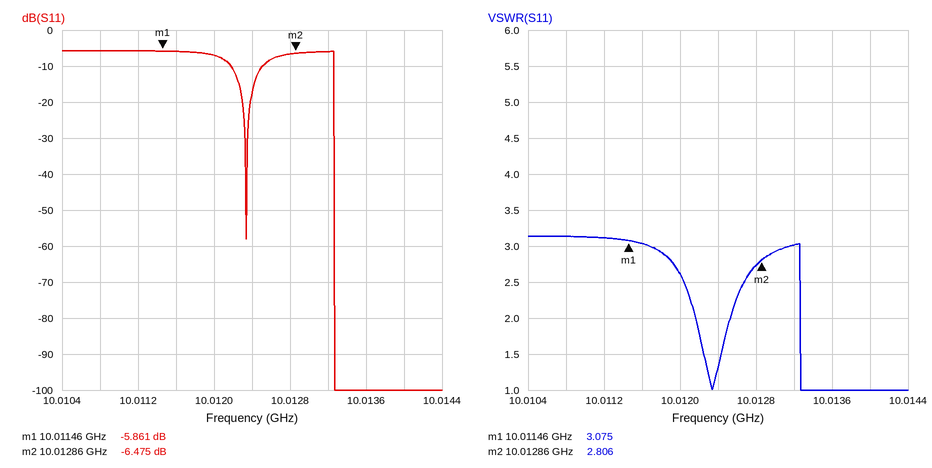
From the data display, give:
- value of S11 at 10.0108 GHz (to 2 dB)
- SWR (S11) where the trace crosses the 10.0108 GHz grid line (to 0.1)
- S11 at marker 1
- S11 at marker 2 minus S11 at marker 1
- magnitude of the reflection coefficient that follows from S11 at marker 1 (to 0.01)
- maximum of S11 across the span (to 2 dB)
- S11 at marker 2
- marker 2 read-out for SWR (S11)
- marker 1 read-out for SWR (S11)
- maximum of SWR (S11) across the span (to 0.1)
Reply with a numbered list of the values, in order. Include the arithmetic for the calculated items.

1. -6 dB
2. 3.1
3. -5.861 dB
4. -6.475 − (-5.861) = -0.614 dB
5. 10^(-5.861/20) ≈ 0.51
6. -6 dB
7. -6.475 dB
8. 2.806
9. 3.075
10. 3.1
